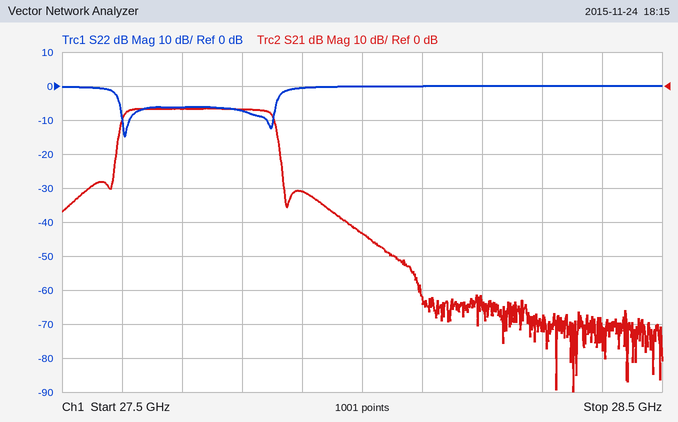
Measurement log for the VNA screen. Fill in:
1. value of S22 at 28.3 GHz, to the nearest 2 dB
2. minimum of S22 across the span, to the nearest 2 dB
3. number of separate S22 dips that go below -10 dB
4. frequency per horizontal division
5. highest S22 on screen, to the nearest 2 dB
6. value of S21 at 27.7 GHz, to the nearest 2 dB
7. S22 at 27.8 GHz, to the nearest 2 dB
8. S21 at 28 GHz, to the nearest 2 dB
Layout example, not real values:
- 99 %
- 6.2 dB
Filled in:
- 0 dB
- -14 dB
- 2
- 100 MHz
- 0 dB
- -6 dB
- -8 dB
- -44 dB
